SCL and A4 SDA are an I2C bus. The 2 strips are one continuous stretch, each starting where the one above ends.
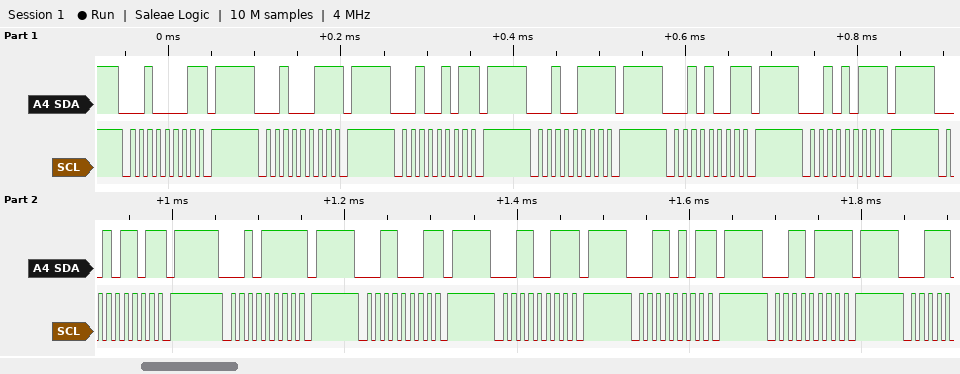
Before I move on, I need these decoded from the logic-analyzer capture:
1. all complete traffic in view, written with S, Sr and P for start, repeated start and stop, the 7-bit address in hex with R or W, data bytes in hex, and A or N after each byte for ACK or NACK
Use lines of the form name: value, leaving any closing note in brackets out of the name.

all complete traffic in view, written with S, Sr and P for start, repeated start and stop, the 7-bit address in hex with R or W, data bytes in hex, and A or N after each byte for ACK or NACK: S 10R N P S 11R N P S 12R N P S 13R N P S 14R N P S 15R N P S 16R N P S 17R N P S 18R N P S 19R N P S 1AR N P S 1BR N P
